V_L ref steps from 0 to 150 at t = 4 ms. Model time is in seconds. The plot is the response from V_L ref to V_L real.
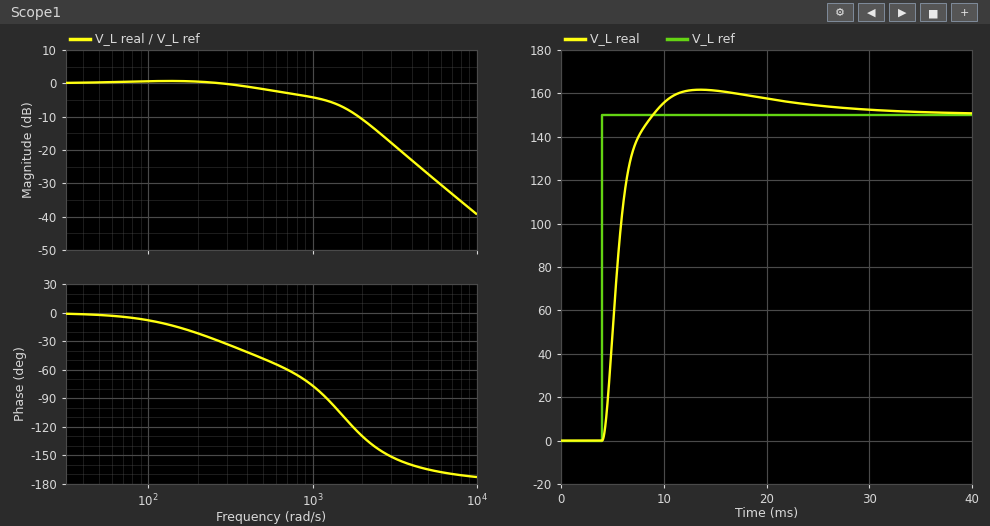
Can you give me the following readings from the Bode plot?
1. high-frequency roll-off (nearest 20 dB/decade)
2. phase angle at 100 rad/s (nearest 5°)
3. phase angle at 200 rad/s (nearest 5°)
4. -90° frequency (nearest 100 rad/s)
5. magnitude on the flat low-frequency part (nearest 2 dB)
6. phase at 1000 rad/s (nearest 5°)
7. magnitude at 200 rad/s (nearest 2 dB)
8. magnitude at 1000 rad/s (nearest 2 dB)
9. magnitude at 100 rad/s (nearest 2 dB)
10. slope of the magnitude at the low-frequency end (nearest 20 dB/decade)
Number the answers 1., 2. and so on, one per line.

1. -40 dB/decade
2. -10°
3. -20°
4. 1200 rad/s
5. 0 dB
6. -75°
7. 0 dB
8. -4 dB
9. 0 dB
10. 0 dB/decade
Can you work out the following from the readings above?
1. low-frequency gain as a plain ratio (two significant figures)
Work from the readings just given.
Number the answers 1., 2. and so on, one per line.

1. 1.0
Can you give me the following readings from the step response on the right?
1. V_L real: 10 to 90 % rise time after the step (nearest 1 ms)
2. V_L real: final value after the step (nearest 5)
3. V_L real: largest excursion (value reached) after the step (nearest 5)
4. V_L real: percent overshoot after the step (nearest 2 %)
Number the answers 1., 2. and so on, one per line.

1. 3 ms
2. 150
3. 160
4. 8 %
